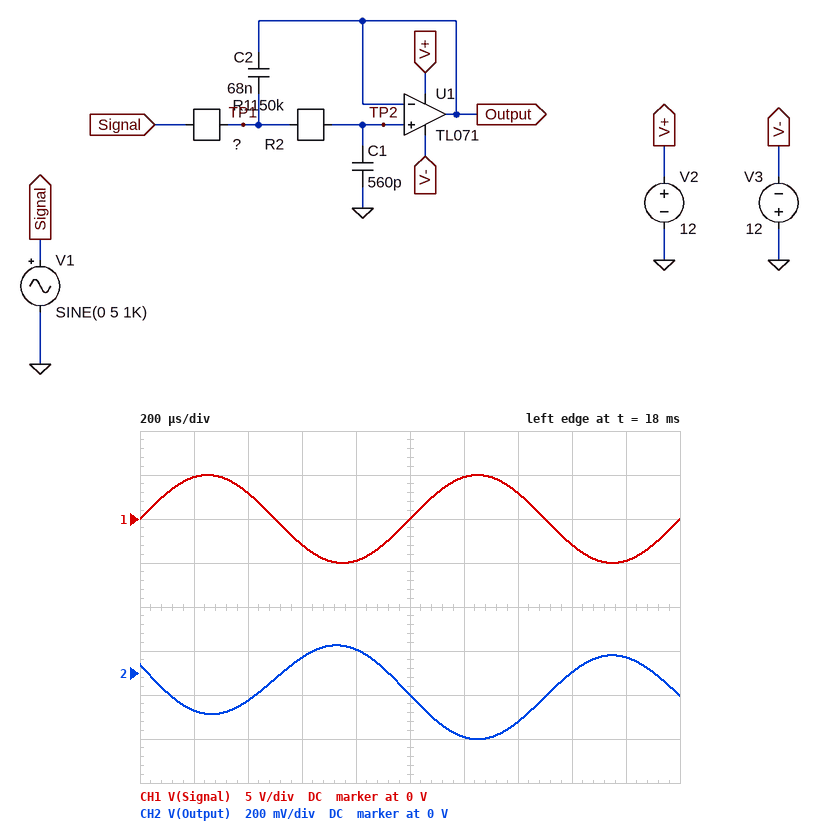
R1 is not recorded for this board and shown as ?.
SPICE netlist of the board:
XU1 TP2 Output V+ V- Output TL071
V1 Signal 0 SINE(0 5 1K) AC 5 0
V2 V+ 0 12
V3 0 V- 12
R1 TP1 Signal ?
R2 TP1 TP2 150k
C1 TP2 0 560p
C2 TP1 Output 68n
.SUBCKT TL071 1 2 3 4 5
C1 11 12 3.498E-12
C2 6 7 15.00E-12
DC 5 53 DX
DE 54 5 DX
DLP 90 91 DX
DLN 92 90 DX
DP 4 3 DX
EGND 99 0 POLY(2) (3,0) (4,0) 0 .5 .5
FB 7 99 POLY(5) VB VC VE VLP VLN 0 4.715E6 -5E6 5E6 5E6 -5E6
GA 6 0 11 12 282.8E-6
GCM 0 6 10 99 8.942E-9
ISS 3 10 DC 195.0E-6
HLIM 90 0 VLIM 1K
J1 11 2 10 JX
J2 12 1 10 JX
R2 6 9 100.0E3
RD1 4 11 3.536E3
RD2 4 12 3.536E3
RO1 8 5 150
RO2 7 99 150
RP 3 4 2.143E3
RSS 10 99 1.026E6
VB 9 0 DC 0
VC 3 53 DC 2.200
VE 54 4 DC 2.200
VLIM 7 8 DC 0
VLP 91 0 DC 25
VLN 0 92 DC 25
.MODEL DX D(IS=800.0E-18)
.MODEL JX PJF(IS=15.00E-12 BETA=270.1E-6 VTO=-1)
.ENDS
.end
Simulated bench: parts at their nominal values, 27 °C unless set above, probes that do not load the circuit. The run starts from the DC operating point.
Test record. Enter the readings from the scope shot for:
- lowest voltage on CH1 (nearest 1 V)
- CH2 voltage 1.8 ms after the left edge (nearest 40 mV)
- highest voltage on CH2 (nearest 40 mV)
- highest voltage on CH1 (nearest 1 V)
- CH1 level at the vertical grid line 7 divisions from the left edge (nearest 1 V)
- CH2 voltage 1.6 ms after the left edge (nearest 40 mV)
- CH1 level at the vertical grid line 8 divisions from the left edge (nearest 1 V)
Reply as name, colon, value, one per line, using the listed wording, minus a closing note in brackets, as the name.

lowest voltage on CH1: -5 V
CH2 voltage 1.8 ms after the left edge: 80 mV
highest voltage on CH2: 120 mV
highest voltage on CH1: 5 V
CH1 level at the vertical grid line 7 divisions from the left edge: 3 V
CH2 voltage 1.6 ms after the left edge: 0 V
CH1 level at the vertical grid line 8 divisions from the left edge: -3 V
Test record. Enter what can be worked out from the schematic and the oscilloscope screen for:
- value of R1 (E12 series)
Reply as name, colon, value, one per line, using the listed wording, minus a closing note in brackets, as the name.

value of R1: 120 kΩ
